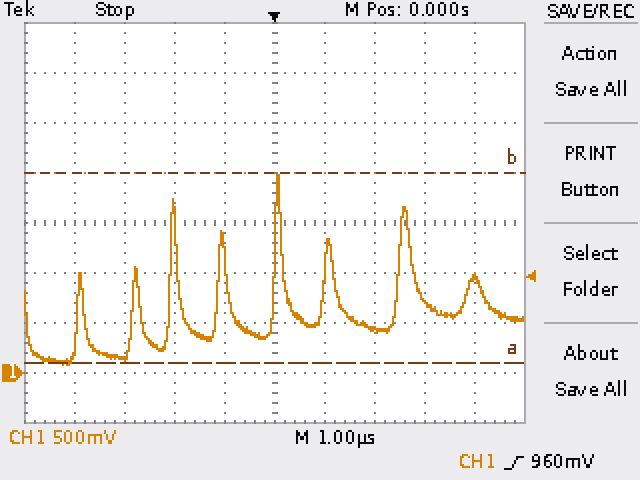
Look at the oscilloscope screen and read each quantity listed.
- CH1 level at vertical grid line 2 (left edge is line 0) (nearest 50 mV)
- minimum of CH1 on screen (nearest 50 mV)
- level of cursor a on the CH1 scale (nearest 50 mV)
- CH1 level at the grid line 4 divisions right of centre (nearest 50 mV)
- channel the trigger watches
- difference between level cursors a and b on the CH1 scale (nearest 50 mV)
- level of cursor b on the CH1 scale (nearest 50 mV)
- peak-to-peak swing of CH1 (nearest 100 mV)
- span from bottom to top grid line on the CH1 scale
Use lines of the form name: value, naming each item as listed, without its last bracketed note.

CH1 level at vertical grid line 2 (left edge is line 0): 150 mV
minimum of CH1 on screen: 100 mV
level of cursor a on the CH1 scale: 100 mV
CH1 level at the grid line 4 divisions right of centre: 950 mV
channel the trigger watches: CH1
difference between level cursors a and b on the CH1 scale: 1.90 V
level of cursor b on the CH1 scale: 2.00 V
peak-to-peak swing of CH1: 1.90 V
span from bottom to top grid line on the CH1 scale: 4 V
